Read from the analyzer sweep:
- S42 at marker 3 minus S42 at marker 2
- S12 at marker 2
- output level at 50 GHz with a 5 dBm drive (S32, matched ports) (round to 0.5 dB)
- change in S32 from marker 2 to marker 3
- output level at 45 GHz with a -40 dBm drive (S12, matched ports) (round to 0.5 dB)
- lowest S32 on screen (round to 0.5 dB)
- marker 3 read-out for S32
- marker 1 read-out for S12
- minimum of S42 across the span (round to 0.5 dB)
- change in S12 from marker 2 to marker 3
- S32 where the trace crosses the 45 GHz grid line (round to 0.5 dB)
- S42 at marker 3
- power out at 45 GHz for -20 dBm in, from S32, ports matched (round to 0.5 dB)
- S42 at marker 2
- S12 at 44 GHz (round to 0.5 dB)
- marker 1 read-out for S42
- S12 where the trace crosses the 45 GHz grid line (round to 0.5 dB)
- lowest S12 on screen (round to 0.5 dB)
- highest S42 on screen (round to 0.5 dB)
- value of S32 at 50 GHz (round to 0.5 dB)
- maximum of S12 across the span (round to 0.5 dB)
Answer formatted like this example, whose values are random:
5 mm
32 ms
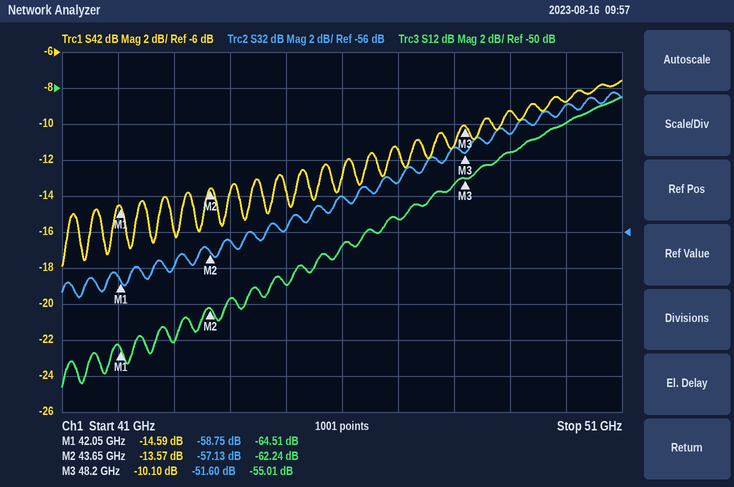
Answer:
3.47 dB
-62.24 dB
-44.0 dBm
5.53 dB
-101.0 dBm
-59.5 dB
-51.60 dB
-64.51 dB
-18.0 dB
7.23 dB
-56.0 dB
-10.10 dB
-76.0 dBm
-13.57 dB
-61.5 dB
-14.59 dB
-61.0 dB
-66.5 dB
-7.5 dB
-49.0 dB
-50.5 dB
